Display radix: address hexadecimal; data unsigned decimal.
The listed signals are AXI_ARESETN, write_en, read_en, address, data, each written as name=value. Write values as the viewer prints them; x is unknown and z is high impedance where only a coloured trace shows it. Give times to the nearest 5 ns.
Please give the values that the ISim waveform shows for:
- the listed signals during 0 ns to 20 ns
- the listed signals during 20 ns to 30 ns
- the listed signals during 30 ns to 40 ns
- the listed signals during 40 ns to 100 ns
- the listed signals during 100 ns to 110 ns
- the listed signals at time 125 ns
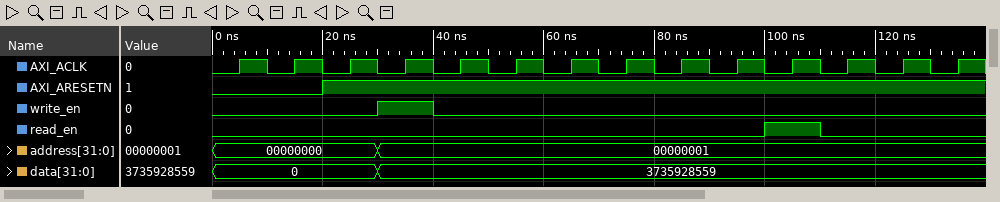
AXI_ARESETN=0, write_en=0, read_en=0, address=00000000, data=0
AXI_ARESETN=1, write_en=0, read_en=0, address=00000000, data=0
AXI_ARESETN=1, write_en=1, read_en=0, address=00000001, data=3735928559
AXI_ARESETN=1, write_en=0, read_en=0, address=00000001, data=3735928559
AXI_ARESETN=1, write_en=0, read_en=1, address=00000001, data=3735928559
AXI_ARESETN=1, write_en=0, read_en=0, address=00000001, data=3735928559
